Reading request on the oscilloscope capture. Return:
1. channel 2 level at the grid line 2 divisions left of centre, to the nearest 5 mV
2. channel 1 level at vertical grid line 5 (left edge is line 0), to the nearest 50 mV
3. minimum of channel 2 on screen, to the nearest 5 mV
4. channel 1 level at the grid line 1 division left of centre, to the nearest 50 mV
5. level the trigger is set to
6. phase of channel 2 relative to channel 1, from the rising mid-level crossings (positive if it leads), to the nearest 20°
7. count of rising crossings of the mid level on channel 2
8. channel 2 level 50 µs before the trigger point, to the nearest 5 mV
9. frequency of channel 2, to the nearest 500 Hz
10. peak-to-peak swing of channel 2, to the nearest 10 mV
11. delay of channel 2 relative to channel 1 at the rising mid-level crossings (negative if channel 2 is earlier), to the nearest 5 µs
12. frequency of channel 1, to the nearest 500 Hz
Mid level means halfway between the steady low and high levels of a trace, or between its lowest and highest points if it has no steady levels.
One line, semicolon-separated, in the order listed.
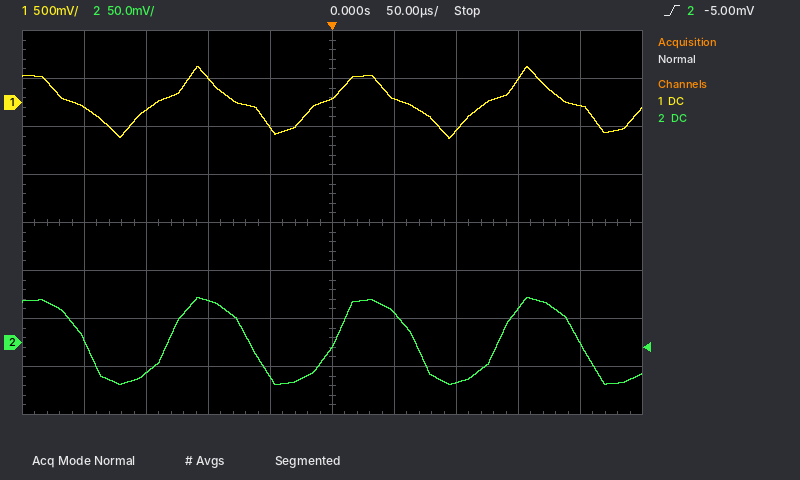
45 mV; 50 mV; -45 mV; -250 mV; -5.00 mV; -20°; 3; -35 mV; 7.5 kHz; 90 mV; +10 µs; 7.5 kHz
